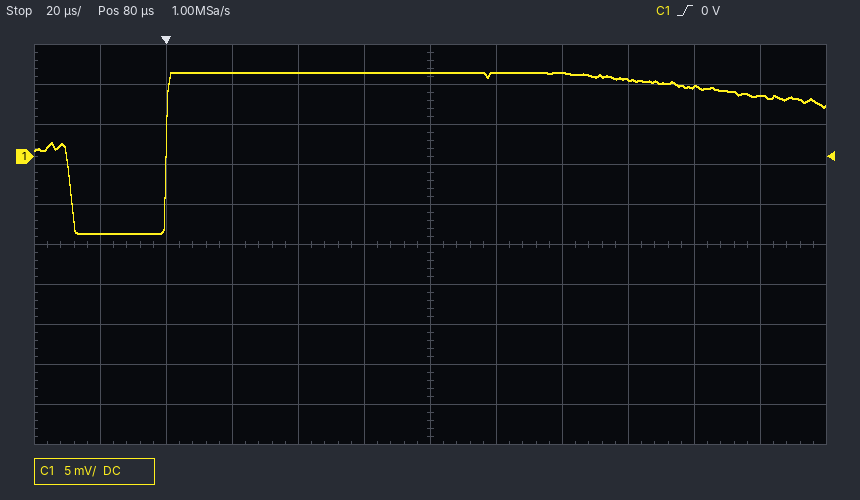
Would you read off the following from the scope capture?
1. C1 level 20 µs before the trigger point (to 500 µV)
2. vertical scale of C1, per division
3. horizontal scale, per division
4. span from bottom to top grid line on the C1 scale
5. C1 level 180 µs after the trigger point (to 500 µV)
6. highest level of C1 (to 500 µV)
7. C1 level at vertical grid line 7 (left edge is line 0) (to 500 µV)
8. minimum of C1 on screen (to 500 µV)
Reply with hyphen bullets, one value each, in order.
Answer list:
- -9.5 mV
- 5 mV
- 20 µs
- 50 mV
- 7.5 mV
- 10.5 mV
- 10.5 mV
- -9.5 mV
